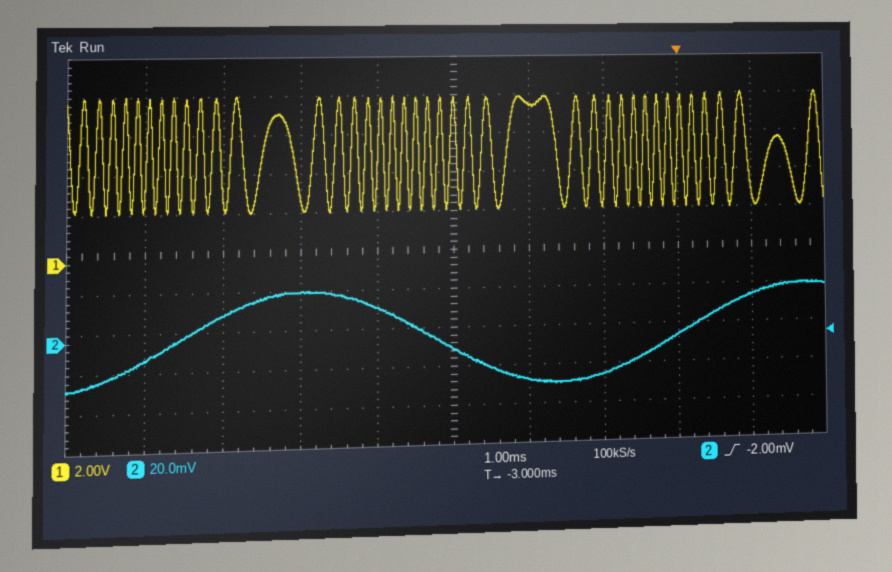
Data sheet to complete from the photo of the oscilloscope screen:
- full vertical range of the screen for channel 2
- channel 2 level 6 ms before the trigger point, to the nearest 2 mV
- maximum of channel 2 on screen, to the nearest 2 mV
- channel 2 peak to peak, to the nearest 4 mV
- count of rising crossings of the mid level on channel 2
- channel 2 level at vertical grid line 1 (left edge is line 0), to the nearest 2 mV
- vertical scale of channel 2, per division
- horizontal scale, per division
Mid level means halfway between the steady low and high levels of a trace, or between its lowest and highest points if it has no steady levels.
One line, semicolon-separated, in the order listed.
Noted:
200 mV; 12 mV; 24 mV; 48 mV; 2; -10 mV; 20 mV; 1 ms
